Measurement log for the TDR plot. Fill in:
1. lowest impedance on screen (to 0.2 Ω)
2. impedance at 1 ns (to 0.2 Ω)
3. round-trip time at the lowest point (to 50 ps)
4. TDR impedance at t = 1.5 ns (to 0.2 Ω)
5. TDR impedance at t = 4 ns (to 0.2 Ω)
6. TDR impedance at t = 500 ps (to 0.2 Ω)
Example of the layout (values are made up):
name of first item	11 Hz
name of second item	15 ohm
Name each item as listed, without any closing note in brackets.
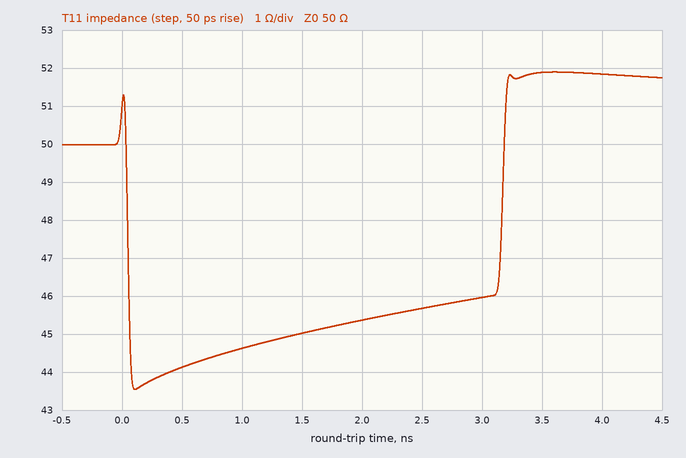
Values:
lowest impedance on screen	43.6 Ω
impedance at 1 ns	44.6 Ω
round-trip time at the lowest point	100 ps
TDR impedance at t = 1.5 ns	45.0 Ω
TDR impedance at t = 4 ns	51.8 Ω
TDR impedance at t = 500 ps	44.2 Ω
